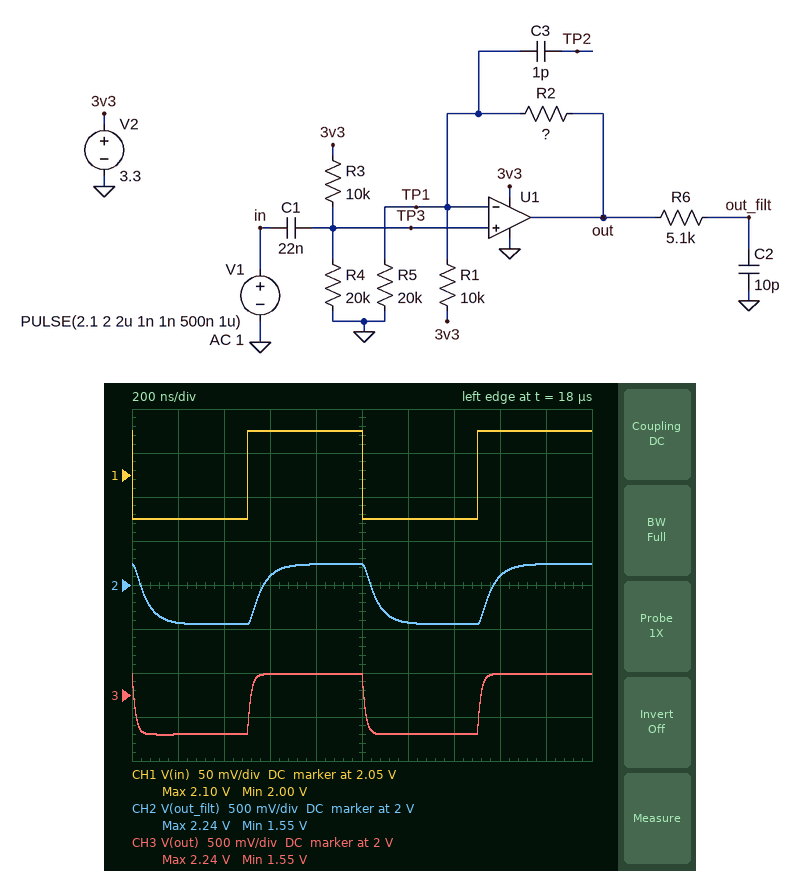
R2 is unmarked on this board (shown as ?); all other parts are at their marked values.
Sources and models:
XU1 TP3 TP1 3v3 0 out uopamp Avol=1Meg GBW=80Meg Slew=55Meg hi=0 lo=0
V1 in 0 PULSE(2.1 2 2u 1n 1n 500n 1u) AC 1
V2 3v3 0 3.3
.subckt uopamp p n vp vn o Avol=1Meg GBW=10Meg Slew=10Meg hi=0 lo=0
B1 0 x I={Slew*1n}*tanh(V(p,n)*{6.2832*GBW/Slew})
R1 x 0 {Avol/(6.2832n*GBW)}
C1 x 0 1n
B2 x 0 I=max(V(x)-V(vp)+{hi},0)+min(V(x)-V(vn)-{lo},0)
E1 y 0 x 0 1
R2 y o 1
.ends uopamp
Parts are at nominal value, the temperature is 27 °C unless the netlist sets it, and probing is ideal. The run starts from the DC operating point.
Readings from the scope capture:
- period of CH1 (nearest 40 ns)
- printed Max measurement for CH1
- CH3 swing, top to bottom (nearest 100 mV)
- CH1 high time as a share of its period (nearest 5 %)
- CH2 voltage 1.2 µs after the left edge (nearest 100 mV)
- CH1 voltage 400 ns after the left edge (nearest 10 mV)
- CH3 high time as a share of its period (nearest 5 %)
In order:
1.00 µs
2.10 V
700 mV
50 %
1.6 V
2.00 V
50 %
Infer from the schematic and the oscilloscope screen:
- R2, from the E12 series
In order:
39 kΩ
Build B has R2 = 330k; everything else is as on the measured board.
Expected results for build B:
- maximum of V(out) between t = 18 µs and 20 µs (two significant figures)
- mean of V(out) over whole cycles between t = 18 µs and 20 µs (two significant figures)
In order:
2.5 V
1.1 V
